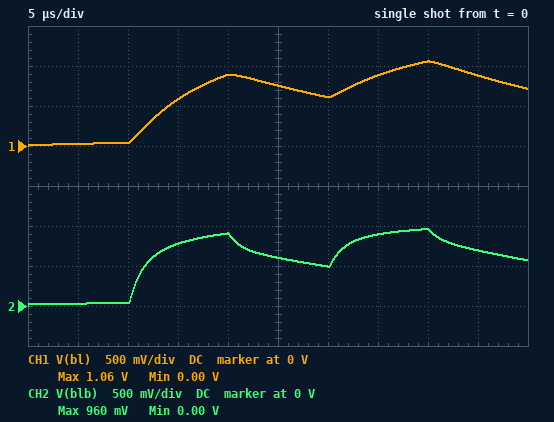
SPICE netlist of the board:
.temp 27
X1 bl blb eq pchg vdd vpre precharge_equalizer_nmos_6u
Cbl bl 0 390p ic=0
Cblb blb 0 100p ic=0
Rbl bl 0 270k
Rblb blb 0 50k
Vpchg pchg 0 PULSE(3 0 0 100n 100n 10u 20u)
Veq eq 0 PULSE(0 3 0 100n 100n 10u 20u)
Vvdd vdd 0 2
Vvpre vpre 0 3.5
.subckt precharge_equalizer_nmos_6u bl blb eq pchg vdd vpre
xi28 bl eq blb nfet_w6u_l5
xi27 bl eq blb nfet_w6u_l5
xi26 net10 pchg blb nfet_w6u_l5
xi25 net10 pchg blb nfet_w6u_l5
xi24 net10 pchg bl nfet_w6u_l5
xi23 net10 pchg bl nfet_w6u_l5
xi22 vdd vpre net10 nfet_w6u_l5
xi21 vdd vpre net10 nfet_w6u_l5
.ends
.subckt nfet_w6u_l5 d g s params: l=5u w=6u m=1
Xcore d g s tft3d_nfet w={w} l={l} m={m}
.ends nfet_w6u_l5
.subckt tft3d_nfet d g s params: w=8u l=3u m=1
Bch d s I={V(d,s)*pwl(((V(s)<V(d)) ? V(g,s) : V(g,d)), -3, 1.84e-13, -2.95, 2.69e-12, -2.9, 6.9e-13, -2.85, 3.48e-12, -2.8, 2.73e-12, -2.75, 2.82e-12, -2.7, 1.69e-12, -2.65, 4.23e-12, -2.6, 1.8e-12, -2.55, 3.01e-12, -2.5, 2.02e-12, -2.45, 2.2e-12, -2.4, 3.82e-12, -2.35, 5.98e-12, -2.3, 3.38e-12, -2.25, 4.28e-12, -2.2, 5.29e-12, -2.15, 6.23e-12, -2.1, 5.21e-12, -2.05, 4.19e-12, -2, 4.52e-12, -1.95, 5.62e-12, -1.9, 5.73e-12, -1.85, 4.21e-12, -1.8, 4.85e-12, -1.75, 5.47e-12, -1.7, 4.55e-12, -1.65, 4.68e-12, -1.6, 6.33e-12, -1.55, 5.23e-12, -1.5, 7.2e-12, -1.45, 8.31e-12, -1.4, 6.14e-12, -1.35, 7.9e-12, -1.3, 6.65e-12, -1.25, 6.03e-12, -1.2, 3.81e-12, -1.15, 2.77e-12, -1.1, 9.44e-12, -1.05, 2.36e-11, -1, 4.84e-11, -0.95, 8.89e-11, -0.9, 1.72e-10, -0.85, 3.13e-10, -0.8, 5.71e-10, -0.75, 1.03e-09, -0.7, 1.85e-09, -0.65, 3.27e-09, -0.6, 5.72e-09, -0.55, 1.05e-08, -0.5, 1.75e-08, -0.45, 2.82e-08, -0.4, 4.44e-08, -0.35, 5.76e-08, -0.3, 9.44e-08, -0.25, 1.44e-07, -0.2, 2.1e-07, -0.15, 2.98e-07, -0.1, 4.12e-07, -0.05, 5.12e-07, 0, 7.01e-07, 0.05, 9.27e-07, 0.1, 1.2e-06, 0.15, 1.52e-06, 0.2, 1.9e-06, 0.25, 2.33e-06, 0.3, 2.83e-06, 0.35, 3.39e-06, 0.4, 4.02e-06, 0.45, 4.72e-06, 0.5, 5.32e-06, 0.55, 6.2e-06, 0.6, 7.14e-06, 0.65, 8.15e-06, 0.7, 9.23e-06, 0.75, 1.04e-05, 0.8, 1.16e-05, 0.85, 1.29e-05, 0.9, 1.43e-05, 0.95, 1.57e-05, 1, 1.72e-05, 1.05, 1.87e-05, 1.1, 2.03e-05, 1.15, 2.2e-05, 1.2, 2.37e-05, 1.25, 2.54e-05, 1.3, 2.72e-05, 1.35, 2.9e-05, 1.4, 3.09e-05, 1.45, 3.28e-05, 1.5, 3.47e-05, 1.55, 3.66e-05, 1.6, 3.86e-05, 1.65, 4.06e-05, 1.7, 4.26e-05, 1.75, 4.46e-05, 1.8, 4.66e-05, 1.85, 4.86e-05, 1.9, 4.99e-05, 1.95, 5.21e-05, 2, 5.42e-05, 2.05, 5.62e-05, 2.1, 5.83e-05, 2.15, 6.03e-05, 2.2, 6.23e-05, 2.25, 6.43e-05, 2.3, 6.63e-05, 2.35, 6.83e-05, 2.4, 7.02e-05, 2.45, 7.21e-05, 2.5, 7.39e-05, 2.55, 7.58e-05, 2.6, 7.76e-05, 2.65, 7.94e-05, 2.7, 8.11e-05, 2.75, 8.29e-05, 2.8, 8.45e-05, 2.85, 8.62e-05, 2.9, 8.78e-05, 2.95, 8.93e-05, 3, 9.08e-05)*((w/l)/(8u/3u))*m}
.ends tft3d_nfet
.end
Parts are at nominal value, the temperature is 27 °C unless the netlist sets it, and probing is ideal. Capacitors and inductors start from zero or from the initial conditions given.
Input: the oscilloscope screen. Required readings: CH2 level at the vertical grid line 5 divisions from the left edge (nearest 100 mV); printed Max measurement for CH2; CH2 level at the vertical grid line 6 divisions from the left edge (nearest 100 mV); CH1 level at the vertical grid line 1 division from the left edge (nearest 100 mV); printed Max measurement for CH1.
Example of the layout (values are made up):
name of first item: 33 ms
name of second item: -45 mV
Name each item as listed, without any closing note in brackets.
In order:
CH2 level at the vertical grid line 5 divisions from the left edge: 600 mV
printed Max measurement for CH2: 960 mV
CH2 level at the vertical grid line 6 divisions from the left edge: 500 mV
CH1 level at the vertical grid line 1 division from the left edge: 0 V
printed Max measurement for CH1: 1.06 V
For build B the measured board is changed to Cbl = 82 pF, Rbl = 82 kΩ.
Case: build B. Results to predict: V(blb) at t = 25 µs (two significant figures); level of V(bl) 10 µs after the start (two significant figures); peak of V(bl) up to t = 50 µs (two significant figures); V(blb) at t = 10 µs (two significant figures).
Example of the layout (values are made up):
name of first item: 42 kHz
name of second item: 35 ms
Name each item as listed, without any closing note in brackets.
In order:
V(blb) at t = 25 µs: 420 mV
level of V(bl) 10 µs after the start: 53 mV
peak of V(bl) up to t = 50 µs: 1.1 V
V(blb) at t = 10 µs: 50 mV
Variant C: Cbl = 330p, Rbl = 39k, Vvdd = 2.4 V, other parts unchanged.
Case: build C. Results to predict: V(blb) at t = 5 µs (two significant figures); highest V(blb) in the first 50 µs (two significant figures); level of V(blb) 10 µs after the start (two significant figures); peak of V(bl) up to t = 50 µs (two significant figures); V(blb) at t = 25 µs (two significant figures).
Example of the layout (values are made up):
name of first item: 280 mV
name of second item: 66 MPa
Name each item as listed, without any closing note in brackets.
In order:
V(blb) at t = 5 µs: 33 mV
highest V(blb) in the first 50 µs: 1.0 V
level of V(blb) 10 µs after the start: 40 mV
peak of V(bl) up to t = 50 µs: 890 mV
V(blb) at t = 25 µs: 480 mV
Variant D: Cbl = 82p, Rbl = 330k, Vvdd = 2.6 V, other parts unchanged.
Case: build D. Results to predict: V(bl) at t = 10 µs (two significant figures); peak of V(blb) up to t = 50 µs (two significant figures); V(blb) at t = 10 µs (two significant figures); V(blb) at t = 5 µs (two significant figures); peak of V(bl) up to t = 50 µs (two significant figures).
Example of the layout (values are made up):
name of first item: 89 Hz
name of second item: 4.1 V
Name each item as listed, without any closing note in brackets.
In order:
V(bl) at t = 10 µs: 81 mV
peak of V(blb) up to t = 50 µs: 1.2 V
V(blb) at t = 10 µs: 73 mV
V(blb) at t = 5 µs: 62 mV
peak of V(bl) up to t = 50 µs: 1.6 V
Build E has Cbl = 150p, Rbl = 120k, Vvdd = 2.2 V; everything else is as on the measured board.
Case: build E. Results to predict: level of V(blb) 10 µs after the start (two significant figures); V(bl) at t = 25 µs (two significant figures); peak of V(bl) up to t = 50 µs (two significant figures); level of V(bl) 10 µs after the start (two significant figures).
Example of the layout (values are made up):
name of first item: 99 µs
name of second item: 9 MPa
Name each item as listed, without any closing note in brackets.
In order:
level of V(blb) 10 µs after the start: 54 mV
V(bl) at t = 25 µs: 700 mV
peak of V(bl) up to t = 50 µs: 1.2 V
level of V(bl) 10 µs after the start: 57 mV
